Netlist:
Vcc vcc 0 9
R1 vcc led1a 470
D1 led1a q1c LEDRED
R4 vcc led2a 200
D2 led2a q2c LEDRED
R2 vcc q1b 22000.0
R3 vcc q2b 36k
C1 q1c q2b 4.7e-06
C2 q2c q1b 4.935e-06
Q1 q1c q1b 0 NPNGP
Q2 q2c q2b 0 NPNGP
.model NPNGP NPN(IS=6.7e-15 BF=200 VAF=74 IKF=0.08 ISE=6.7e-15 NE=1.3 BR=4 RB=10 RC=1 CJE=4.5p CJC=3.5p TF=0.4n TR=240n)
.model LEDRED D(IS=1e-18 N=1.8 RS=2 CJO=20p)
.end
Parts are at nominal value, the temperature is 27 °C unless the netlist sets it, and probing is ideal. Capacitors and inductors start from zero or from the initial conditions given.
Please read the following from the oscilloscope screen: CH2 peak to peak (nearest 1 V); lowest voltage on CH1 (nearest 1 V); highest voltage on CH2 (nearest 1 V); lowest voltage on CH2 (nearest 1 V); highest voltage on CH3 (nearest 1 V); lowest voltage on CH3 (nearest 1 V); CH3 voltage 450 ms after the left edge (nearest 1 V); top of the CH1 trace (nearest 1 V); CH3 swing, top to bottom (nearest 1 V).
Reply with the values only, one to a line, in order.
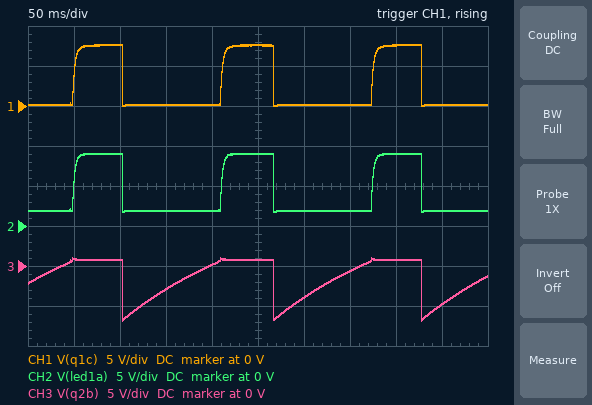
7 V
0 V
9 V
2 V
1 V
-7 V
-5 V
8 V
8 V
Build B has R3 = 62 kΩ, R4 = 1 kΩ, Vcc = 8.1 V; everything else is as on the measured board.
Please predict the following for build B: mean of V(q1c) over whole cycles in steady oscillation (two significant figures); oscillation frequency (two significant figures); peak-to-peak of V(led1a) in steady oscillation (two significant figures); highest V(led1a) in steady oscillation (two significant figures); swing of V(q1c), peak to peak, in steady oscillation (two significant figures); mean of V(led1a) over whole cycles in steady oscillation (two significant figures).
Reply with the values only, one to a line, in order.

1.8 V
4.0 Hz
6.3 V
8.1 V
6.7 V
3.5 V
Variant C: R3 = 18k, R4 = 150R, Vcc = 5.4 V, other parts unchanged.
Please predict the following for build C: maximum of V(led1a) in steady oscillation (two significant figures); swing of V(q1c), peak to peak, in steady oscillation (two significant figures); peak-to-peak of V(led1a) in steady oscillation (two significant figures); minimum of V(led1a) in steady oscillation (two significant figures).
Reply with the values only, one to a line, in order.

5.4 V
4.0 V
3.7 V
1.7 V
